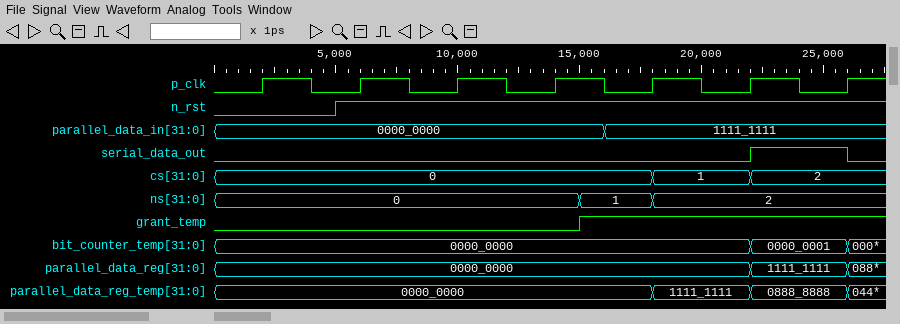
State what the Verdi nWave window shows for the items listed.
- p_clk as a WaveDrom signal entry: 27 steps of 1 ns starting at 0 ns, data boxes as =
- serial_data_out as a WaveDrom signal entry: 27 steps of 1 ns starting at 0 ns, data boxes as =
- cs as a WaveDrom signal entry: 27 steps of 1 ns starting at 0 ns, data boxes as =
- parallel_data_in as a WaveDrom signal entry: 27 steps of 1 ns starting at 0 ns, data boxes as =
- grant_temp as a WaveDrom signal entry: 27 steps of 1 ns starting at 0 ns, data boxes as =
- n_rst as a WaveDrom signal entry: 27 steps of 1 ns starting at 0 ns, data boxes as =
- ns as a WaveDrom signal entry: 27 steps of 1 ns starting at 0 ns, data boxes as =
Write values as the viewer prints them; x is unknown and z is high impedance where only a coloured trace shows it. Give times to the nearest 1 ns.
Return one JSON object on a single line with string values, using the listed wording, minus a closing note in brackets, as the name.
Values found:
{"p_clk as a WaveDrom signal entry: 27 steps of 1 ns starting at 0 ns, data boxes as =": "{name: 'p_clk', wave: '0.1.0.1.0.1.0.1.0.1.0.1.0.1'}", "serial_data_out as a WaveDrom signal entry: 27 steps of 1 ns starting at 0 ns, data boxes as =": "{name: 'serial_data_out', wave: '0.....................1...0'}", "cs as a WaveDrom signal entry: 27 steps of 1 ns starting at 0 ns, data boxes as =": "{name: 'cs', wave: '=.................=...=....', data: '0 1 2'}", "parallel_data_in as a WaveDrom signal entry: 27 steps of 1 ns starting at 0 ns, data boxes as =": "{name: 'parallel_data_in', wave: '=...............=..........', data: '0000_0000 1111_1111'}", "grant_temp as a WaveDrom signal entry: 27 steps of 1 ns starting at 0 ns, data boxes as =": "{name: 'grant_temp', wave: '0..............1...........'}", "n_rst as a WaveDrom signal entry: 27 steps of 1 ns starting at 0 ns, data boxes as =": "{name: 'n_rst', wave: '0....1.....................'}", "ns as a WaveDrom signal entry: 27 steps of 1 ns starting at 0 ns, data boxes as =": "{name: 'ns', wave: '=..............=..=........', data: '0 1 2'}"}
